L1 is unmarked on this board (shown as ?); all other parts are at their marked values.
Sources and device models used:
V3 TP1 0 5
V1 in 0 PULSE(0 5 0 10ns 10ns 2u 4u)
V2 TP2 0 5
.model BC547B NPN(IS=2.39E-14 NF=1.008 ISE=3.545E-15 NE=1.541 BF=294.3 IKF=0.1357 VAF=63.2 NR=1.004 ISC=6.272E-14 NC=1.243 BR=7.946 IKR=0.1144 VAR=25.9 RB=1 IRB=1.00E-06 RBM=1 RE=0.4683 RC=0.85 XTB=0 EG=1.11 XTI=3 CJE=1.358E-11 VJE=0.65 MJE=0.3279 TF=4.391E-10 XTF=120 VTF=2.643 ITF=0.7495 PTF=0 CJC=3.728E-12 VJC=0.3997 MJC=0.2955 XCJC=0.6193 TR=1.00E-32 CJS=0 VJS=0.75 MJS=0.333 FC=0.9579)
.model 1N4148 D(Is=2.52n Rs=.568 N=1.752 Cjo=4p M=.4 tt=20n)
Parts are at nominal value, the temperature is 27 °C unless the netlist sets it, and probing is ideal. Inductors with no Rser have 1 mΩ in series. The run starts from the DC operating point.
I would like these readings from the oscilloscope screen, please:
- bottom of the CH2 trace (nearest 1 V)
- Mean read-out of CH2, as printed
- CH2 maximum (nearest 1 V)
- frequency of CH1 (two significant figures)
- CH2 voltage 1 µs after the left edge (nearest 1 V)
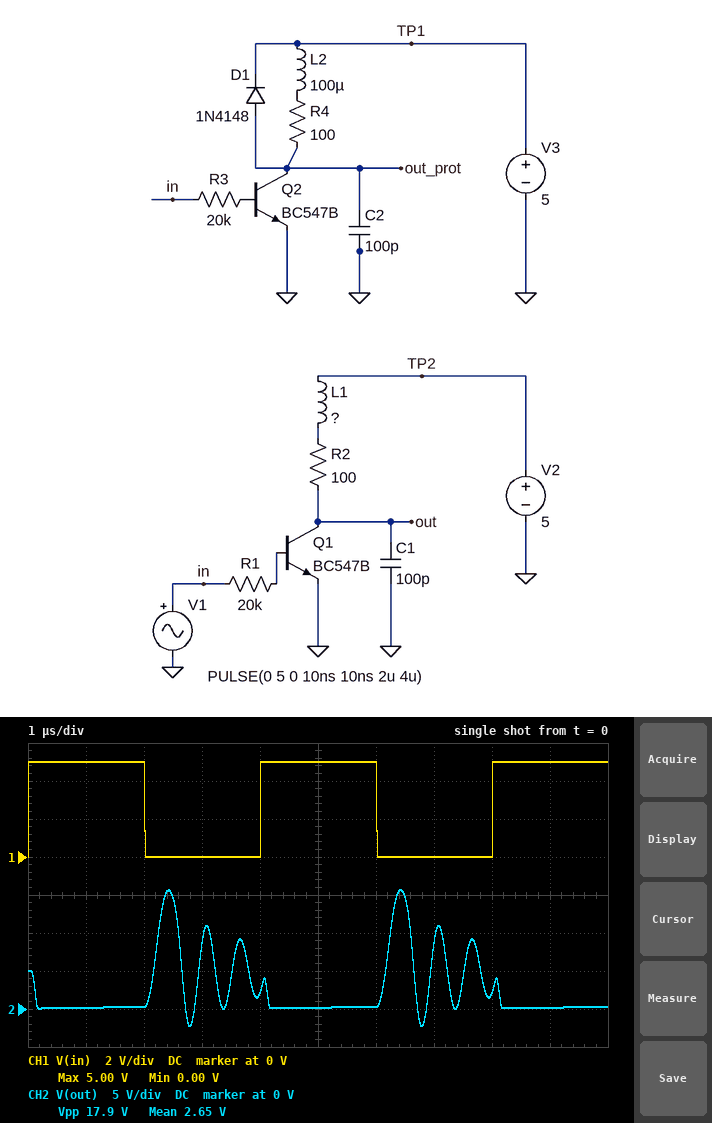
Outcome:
-2 V
2.65 V
16 V
250 kHz
0 V
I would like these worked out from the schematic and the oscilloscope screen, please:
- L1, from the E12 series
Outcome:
82 µH
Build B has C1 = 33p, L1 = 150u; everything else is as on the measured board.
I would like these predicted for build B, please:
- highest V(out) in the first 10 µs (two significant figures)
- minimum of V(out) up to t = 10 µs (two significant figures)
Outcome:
20 V
-3.8 V
